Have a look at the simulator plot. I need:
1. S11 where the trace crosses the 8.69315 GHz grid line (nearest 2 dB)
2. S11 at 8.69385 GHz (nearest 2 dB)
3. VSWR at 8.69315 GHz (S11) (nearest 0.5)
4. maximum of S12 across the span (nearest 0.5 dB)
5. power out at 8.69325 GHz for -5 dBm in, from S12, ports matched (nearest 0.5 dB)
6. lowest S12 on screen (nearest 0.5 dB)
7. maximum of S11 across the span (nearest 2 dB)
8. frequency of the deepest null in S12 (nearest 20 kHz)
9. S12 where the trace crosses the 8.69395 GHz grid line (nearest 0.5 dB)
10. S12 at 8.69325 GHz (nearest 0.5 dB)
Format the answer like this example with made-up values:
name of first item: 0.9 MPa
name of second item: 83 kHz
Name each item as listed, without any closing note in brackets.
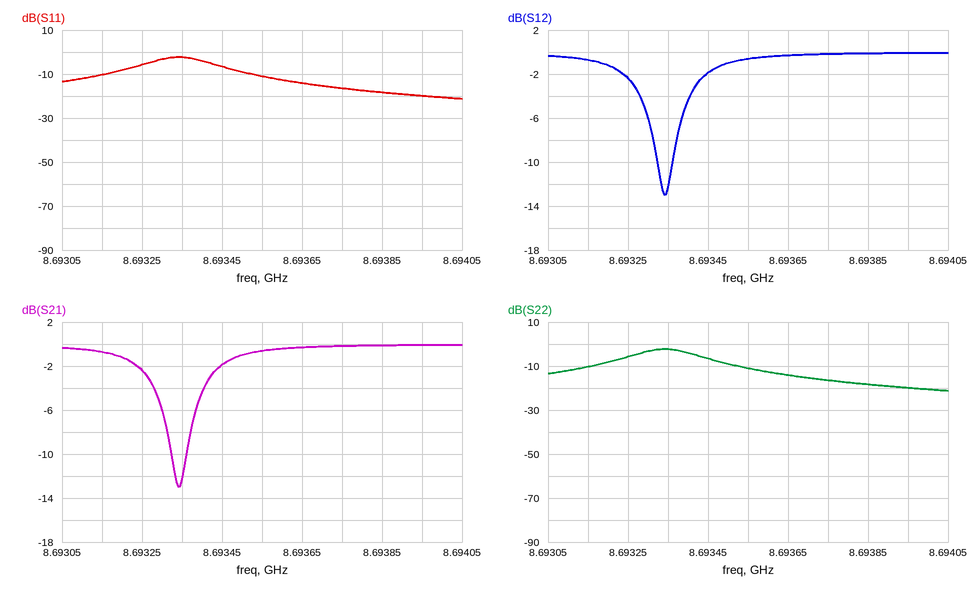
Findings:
S11 where the trace crosses the 8.69315 GHz grid line: -10 dB
S11 at 8.69385 GHz: -18 dB
VSWR at 8.69315 GHz (S11): 2.0
maximum of S12 across the span: 0.0 dB
power out at 8.69325 GHz for -5 dBm in, from S12, ports matched: -7.5 dBm
lowest S12 on screen: -13.0 dB
maximum of S11 across the span: -2 dB
frequency of the deepest null in S12: 8.69334 GHz
S12 where the trace crosses the 8.69395 GHz grid line: 0.0 dB
S12 at 8.69325 GHz: -2.5 dB
